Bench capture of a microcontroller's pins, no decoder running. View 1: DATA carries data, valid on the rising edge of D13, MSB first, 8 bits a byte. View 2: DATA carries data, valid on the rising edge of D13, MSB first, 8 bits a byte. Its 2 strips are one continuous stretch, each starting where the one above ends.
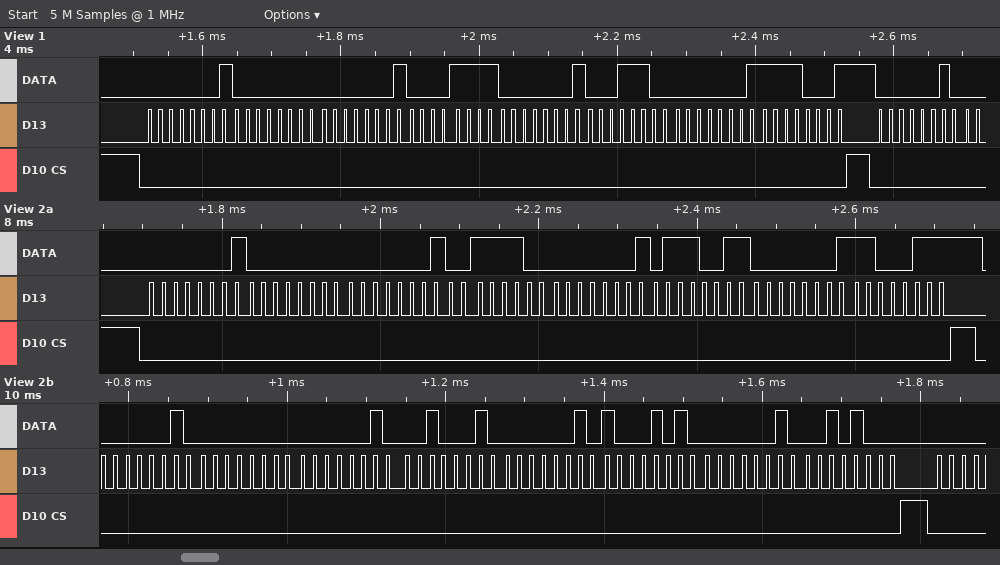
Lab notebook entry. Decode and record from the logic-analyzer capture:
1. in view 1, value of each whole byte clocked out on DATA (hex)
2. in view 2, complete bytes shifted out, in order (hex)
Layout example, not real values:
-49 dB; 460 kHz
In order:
0x01 0x00 0x01 0x0F 0x01 0x1C 0x01 0xF1 0x02; 0x01 0x00 0x01 0x3C 0x01 0x73 0x01 0xC7 0x02 0x00 0x02 0x22 0x02 0x8A 0x02 0x28
